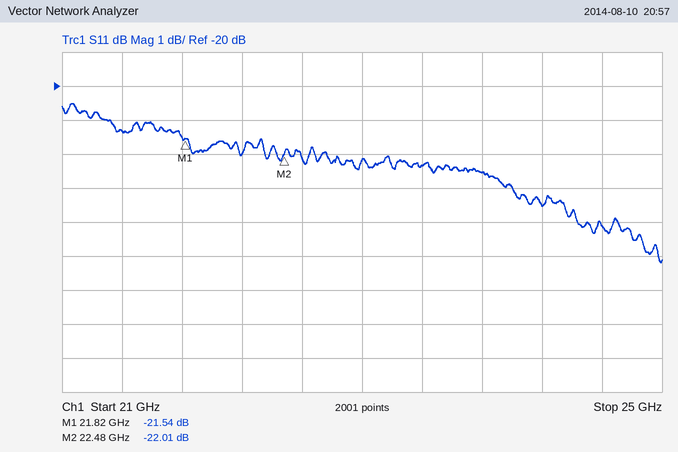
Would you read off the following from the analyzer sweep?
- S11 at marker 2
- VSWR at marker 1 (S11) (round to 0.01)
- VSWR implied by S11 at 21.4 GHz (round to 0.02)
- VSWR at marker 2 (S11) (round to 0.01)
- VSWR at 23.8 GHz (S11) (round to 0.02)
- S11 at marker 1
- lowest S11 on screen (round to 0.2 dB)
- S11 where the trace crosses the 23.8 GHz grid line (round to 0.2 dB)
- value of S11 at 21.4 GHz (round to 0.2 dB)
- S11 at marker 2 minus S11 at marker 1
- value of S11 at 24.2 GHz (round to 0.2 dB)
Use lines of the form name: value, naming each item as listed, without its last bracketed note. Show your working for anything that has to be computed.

S11 at marker 2: -22.01 dB
VSWR at marker 1 (S11): (1 + 0.0838)/(1 − 0.0838) ≈ 1.18
VSWR implied by S11 at 21.4 GHz: |Γ| = 10^(-21.4/20) = 0.0851; VSWR = (1 + 0.0851)/(1 − 0.0851) ≈ 1.19, so 1.18 to the nearest 0.02
VSWR at marker 2 (S11): (1 + 0.0793)/(1 − 0.0793) ≈ 1.17
VSWR at 23.8 GHz (S11): |Γ| = 10^(-22.6/20) = 0.0741; VSWR = (1 + 0.0741)/(1 − 0.0741) ≈ 1.16
S11 at marker 1: -21.54 dB
lowest S11 on screen: -25.2 dB
S11 where the trace crosses the 23.8 GHz grid line: -22.6 dB
value of S11 at 21.4 GHz: -21.4 dB
S11 at marker 2 minus S11 at marker 1: -22.01 − (-21.54) = -0.47 dB
value of S11 at 24.2 GHz: -23.6 dB
